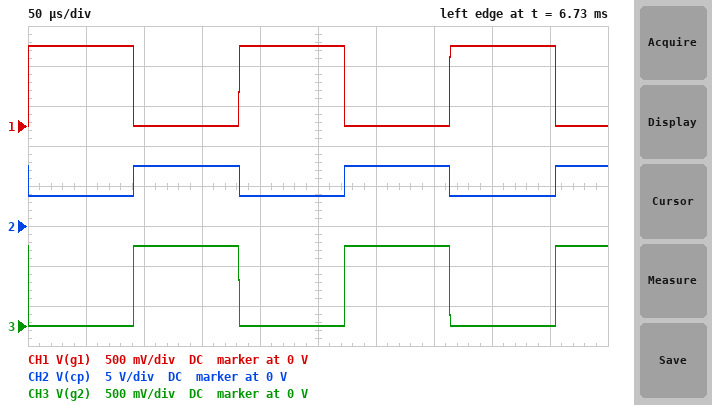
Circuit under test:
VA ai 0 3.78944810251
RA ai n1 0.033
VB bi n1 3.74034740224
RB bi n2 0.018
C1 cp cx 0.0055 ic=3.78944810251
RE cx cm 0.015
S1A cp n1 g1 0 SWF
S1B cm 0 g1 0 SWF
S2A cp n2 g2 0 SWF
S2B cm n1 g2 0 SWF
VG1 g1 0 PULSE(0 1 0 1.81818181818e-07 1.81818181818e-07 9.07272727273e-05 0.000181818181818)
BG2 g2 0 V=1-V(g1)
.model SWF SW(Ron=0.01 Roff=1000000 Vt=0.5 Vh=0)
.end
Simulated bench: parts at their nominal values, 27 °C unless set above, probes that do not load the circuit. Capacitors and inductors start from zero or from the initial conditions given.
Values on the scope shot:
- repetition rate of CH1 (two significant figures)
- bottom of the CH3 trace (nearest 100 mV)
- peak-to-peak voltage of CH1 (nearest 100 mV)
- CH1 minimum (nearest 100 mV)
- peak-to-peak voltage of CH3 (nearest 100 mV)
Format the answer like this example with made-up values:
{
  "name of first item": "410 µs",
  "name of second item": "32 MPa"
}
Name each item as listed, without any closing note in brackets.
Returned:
{
  "repetition rate of CH1": "5.5 kHz",
  "bottom of the CH3 trace": "0 V",
  "peak-to-peak voltage of CH1": "1.0 V",
  "CH1 minimum": "0 V",
  "peak-to-peak voltage of CH3": "1.0 V"
}
